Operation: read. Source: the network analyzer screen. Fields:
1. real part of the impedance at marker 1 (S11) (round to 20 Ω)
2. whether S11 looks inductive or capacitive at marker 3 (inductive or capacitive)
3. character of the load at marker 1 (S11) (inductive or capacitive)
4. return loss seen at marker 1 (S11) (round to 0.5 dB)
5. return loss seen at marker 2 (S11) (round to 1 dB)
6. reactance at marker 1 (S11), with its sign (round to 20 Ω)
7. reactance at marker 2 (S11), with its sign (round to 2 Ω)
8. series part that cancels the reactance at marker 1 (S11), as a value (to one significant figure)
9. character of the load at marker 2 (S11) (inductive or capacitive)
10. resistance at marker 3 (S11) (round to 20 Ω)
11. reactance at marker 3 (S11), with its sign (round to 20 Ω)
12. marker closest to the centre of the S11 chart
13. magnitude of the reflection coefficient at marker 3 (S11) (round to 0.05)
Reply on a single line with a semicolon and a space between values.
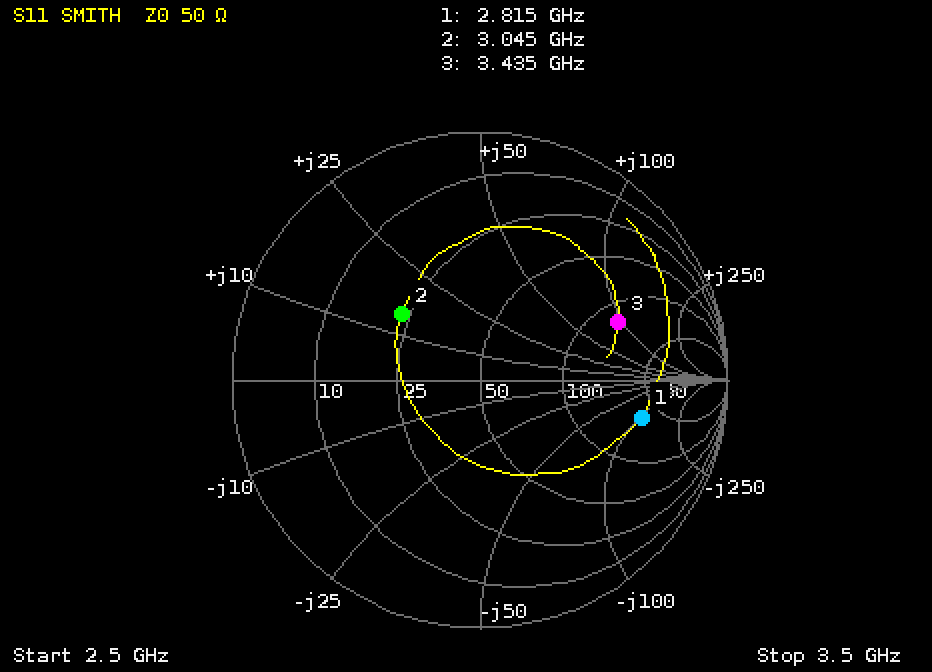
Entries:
200 Ω; inductive; capacitive; 3.5 dB; 8 dB; -100 Ω; +14 Ω; 6 nH; inductive; 120 Ω; +100 Ω; marker 2; 0.60
